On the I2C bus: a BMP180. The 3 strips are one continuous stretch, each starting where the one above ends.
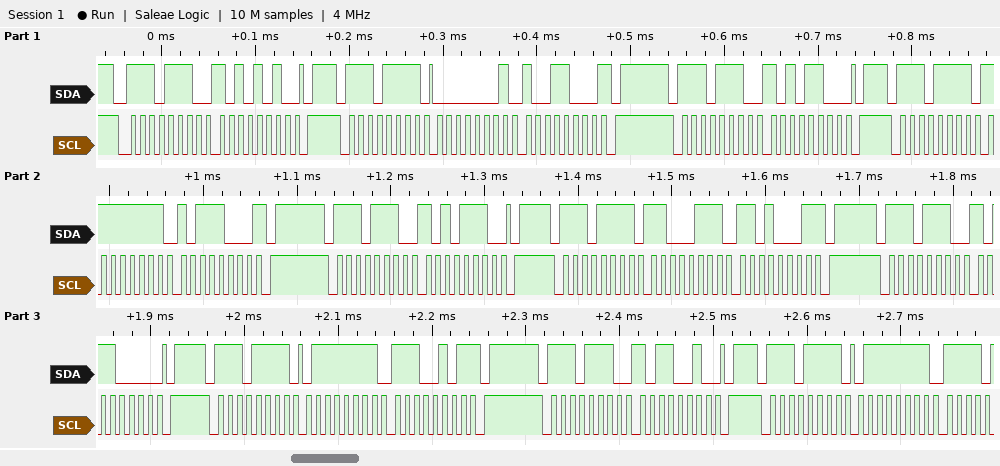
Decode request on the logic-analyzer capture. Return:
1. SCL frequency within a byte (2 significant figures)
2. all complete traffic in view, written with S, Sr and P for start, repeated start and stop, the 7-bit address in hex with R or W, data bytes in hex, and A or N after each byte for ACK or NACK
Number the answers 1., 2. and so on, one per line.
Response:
1. 100 kHz
2. S 77W A AA A P S 77R A 01 A 98 N P S 77W A AC A P S 77R A FF A B8 N P S 77W A AE A P S 77R A C7 A D1 N P S 77W A B0 A P S 77R A 7F A E5 N P S 77W A B2 A P S 77R A 7F A
